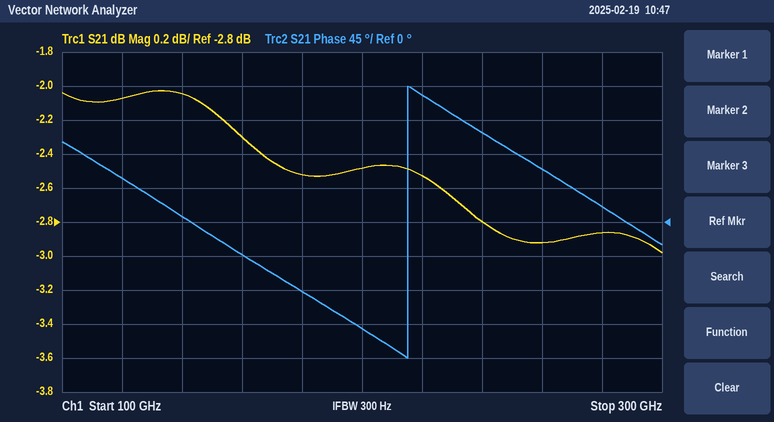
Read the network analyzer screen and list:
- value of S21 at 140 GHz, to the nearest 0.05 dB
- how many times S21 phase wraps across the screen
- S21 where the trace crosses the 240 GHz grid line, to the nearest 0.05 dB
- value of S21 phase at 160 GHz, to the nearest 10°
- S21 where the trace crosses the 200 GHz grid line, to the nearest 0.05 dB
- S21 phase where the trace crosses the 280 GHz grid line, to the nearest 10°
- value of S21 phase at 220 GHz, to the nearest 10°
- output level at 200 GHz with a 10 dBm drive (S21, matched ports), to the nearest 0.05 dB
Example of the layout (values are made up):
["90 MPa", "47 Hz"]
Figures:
["-2.05 dB", "1", "-2.80 dB", "-40°", "-2.50 dB", "20°", "170°", "7.50 dBm"]
